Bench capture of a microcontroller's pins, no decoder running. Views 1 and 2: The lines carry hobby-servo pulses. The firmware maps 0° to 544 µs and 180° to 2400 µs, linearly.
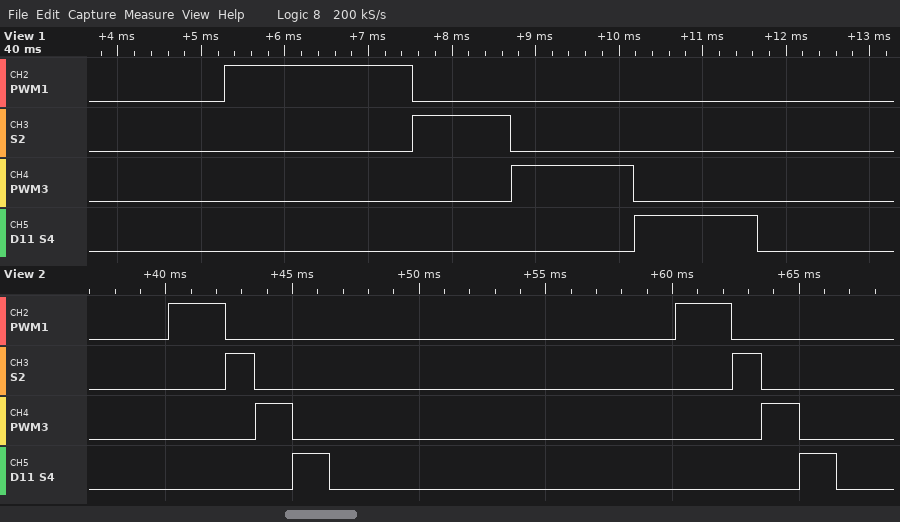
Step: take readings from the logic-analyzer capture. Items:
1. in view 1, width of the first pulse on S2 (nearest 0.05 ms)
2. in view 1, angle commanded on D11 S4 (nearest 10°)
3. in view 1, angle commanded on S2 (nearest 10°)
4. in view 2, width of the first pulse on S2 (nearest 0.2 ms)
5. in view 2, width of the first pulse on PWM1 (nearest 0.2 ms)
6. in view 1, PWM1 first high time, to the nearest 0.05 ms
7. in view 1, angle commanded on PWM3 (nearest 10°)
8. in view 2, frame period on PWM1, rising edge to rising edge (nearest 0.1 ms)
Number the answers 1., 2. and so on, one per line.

1. 1.15 ms
2. 90°
3. 60°
4. 1.2 ms
5. 2.2 ms
6. 2.25 ms
7. 90°
8. 20.0 ms
